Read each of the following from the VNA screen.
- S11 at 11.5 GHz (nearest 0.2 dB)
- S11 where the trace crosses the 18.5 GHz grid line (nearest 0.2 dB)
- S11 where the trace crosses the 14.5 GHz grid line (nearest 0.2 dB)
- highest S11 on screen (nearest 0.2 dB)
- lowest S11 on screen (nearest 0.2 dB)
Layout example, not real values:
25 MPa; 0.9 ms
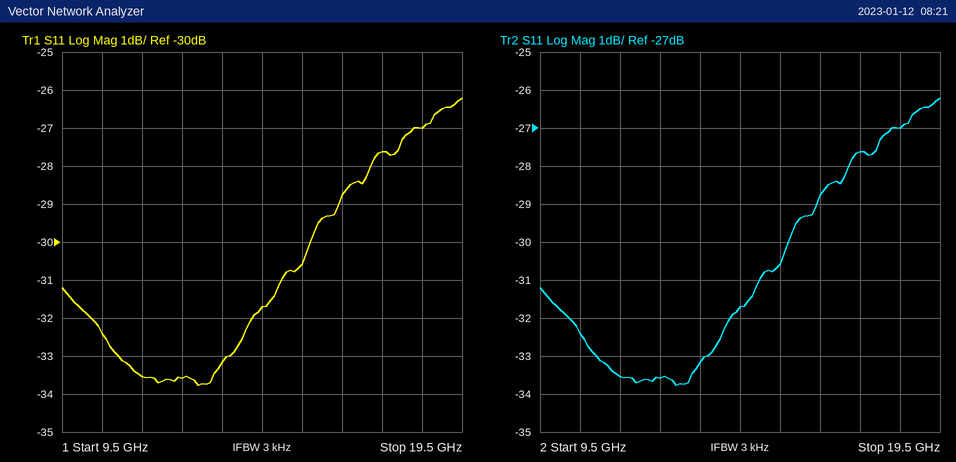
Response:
-33.6 dB; -27.0 dB; -31.8 dB; -26.2 dB; -33.8 dB
